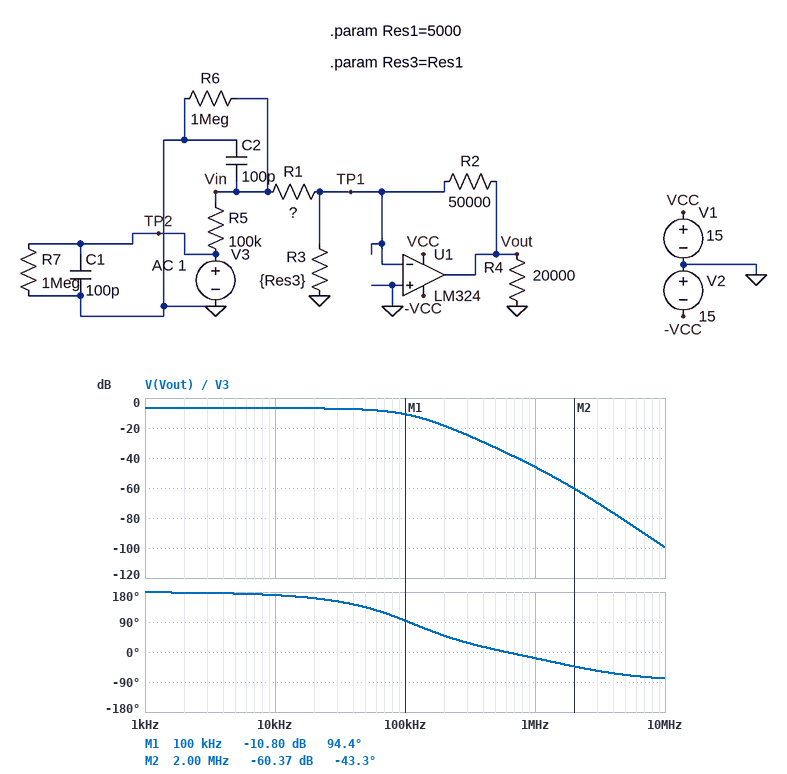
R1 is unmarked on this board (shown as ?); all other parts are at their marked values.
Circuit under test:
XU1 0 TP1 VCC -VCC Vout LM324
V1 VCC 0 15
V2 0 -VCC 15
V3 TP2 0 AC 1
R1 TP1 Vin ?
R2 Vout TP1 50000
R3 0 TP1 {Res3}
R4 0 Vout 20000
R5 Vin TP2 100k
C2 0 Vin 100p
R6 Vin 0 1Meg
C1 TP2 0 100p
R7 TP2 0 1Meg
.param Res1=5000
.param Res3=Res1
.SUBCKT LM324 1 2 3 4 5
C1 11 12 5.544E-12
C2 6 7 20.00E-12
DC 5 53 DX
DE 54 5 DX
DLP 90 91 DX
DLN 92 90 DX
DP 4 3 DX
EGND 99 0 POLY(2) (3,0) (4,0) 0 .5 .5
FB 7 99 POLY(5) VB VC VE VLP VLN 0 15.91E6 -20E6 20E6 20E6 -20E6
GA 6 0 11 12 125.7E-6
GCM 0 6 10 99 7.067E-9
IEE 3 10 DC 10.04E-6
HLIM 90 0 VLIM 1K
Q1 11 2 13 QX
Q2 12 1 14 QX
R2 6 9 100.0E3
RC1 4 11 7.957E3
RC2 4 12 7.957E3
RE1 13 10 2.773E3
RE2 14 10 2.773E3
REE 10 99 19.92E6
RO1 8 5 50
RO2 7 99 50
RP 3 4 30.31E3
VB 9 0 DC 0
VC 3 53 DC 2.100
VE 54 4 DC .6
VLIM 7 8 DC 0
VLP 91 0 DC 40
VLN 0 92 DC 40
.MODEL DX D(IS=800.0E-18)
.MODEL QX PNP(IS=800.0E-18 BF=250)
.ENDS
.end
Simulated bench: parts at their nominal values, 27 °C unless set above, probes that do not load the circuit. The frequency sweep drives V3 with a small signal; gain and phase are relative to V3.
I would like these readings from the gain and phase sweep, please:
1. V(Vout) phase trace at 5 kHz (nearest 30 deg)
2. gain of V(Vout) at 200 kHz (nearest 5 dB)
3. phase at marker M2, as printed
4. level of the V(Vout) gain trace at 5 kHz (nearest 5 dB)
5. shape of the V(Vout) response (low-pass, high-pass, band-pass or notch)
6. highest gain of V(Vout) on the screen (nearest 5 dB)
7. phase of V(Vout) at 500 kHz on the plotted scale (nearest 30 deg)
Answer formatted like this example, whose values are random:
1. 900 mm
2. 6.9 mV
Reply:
1. 180 deg
2. -20 dB
3. -43.3 deg
4. -5 dB
5. low-pass
6. -5 dB
7. 0 deg
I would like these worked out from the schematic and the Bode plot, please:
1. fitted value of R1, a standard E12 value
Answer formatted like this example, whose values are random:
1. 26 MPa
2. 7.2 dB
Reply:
1. 8.2 kΩ
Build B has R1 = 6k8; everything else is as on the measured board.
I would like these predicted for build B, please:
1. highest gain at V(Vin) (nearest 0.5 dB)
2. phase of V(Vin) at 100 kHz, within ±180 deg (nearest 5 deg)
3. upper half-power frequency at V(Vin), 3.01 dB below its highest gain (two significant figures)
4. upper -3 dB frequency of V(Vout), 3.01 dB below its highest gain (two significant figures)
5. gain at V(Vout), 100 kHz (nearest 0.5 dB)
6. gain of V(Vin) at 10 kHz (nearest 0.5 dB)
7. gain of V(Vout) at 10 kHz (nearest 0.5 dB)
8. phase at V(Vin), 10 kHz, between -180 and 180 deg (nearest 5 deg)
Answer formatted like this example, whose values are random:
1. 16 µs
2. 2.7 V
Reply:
1. -21.5 dB
2. -20 deg
3. 230 kHz
4. 90 kHz
5. -10.5 dB
6. -24.0 dB
7. -6.5 dB
8. 0 deg
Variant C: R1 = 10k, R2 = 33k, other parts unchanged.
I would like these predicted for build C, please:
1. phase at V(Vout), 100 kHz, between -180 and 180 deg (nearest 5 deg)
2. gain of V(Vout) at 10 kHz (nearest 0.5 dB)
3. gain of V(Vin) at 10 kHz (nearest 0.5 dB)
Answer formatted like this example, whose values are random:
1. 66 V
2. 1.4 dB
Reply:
1. 105 deg
2. -10.5 dB
3. -21.0 dB
